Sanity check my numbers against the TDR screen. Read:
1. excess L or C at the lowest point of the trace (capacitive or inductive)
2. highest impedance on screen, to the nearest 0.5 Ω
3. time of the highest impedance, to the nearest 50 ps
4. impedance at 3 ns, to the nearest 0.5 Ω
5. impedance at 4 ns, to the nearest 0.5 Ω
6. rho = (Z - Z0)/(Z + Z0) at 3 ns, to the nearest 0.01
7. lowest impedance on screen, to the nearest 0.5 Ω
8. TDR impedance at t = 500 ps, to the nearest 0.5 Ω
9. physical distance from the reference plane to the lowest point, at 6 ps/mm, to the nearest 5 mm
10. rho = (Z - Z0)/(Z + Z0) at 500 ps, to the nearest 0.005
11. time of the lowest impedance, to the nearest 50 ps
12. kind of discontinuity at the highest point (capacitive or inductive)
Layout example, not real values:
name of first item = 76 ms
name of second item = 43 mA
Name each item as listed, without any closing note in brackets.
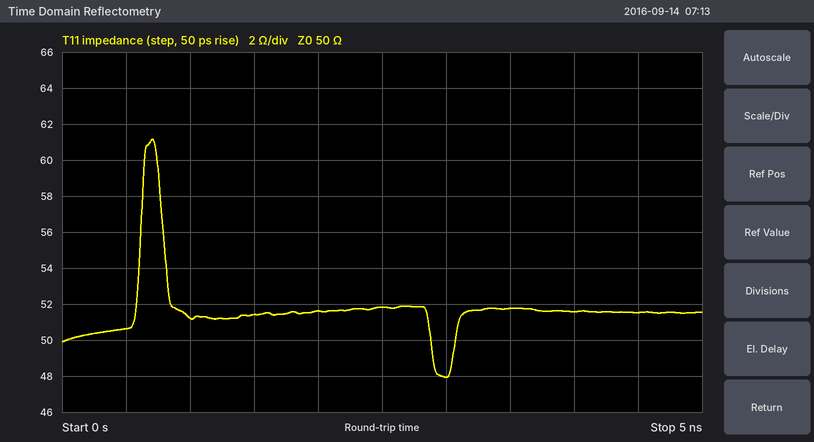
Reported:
excess L or C at the lowest point of the trace = capacitive
highest impedance on screen, to the nearest 0.5 Ω = 61.0 Ω
time of the highest impedance, to the nearest 50 ps = 700 ps
impedance at 3 ns, to the nearest 0.5 Ω = 48.0 Ω
impedance at 4 ns, to the nearest 0.5 Ω = 51.5 Ω
rho = (Z - Z0)/(Z + Z0) at 3 ns, to the nearest 0.01 = -0.02
lowest impedance on screen, to the nearest 0.5 Ω = 48.0 Ω
TDR impedance at t = 500 ps, to the nearest 0.5 Ω = 50.5 Ω
physical distance from the reference plane to the lowest point, at 6 ps/mm, to the nearest 5 mm = 250 mm
rho = (Z - Z0)/(Z + Z0) at 500 ps, to the nearest 0.005 = +0.005
time of the lowest impedance, to the nearest 50 ps = 3.00 ns
kind of discontinuity at the highest point = inductive
